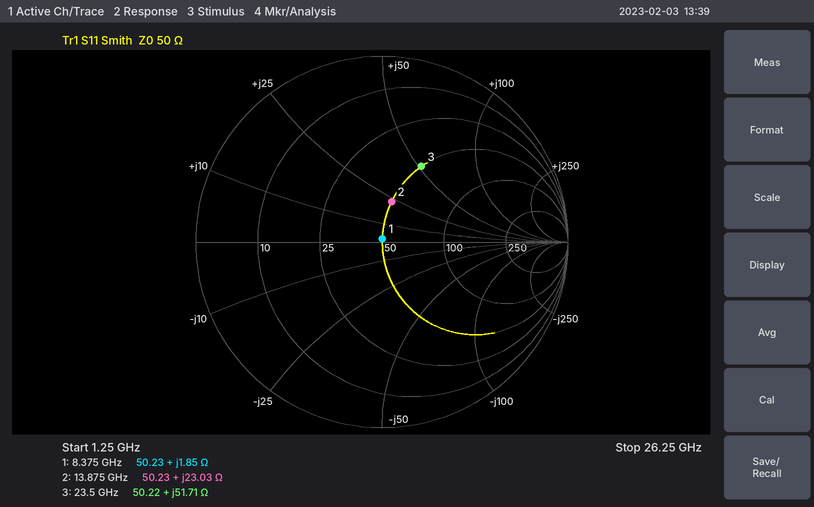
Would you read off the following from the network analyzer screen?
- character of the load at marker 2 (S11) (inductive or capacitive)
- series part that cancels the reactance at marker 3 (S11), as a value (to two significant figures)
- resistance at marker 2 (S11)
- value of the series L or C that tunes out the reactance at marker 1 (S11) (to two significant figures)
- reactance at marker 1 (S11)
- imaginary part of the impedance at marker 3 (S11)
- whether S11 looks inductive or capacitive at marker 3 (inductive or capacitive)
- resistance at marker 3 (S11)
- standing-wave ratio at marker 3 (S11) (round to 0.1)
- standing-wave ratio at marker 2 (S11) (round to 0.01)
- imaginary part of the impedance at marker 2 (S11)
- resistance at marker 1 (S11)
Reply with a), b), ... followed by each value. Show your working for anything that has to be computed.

a) inductive
b) C = 1/(2π × 23.5 GHz × 51.71 Ω) ≈ 131 fF, so 130 fF to two significant figures
c) 50.23 Ω
d) C = 1/(2π × 8.375 GHz × 1.85 Ω) ≈ 10 pF
e) +1.85 Ω
f) +51.71 Ω
g) inductive
h) 50.22 Ω
i) 2.7
j) 1.58
k) +23.03 Ω
l) 50.23 Ω
